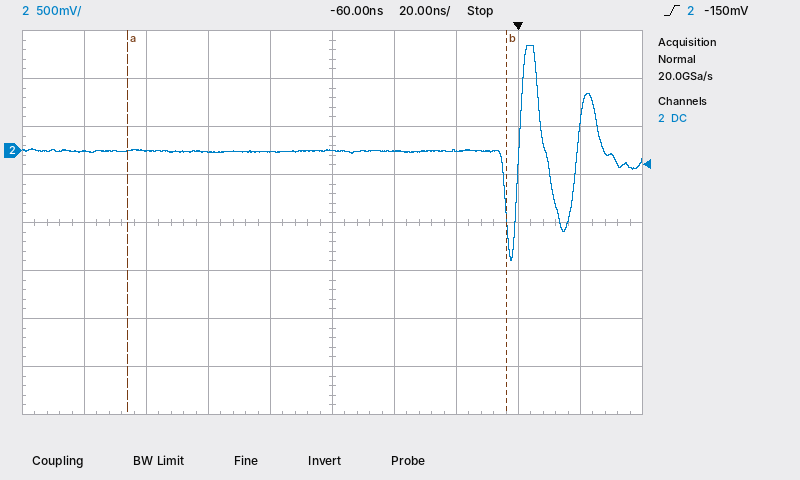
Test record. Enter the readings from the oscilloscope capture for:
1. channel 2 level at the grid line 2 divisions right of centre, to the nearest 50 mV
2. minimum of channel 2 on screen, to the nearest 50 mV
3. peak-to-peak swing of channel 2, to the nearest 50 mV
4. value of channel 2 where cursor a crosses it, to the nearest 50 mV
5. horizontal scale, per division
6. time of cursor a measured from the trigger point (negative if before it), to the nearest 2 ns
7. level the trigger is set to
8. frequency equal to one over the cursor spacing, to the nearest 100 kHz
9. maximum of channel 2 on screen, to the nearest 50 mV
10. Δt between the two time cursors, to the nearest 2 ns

0 mV
-1.15 V
2.25 V
0 mV
20 ns
-126 ns
-150 mV
8.2 MHz
1.10 V
122 ns
